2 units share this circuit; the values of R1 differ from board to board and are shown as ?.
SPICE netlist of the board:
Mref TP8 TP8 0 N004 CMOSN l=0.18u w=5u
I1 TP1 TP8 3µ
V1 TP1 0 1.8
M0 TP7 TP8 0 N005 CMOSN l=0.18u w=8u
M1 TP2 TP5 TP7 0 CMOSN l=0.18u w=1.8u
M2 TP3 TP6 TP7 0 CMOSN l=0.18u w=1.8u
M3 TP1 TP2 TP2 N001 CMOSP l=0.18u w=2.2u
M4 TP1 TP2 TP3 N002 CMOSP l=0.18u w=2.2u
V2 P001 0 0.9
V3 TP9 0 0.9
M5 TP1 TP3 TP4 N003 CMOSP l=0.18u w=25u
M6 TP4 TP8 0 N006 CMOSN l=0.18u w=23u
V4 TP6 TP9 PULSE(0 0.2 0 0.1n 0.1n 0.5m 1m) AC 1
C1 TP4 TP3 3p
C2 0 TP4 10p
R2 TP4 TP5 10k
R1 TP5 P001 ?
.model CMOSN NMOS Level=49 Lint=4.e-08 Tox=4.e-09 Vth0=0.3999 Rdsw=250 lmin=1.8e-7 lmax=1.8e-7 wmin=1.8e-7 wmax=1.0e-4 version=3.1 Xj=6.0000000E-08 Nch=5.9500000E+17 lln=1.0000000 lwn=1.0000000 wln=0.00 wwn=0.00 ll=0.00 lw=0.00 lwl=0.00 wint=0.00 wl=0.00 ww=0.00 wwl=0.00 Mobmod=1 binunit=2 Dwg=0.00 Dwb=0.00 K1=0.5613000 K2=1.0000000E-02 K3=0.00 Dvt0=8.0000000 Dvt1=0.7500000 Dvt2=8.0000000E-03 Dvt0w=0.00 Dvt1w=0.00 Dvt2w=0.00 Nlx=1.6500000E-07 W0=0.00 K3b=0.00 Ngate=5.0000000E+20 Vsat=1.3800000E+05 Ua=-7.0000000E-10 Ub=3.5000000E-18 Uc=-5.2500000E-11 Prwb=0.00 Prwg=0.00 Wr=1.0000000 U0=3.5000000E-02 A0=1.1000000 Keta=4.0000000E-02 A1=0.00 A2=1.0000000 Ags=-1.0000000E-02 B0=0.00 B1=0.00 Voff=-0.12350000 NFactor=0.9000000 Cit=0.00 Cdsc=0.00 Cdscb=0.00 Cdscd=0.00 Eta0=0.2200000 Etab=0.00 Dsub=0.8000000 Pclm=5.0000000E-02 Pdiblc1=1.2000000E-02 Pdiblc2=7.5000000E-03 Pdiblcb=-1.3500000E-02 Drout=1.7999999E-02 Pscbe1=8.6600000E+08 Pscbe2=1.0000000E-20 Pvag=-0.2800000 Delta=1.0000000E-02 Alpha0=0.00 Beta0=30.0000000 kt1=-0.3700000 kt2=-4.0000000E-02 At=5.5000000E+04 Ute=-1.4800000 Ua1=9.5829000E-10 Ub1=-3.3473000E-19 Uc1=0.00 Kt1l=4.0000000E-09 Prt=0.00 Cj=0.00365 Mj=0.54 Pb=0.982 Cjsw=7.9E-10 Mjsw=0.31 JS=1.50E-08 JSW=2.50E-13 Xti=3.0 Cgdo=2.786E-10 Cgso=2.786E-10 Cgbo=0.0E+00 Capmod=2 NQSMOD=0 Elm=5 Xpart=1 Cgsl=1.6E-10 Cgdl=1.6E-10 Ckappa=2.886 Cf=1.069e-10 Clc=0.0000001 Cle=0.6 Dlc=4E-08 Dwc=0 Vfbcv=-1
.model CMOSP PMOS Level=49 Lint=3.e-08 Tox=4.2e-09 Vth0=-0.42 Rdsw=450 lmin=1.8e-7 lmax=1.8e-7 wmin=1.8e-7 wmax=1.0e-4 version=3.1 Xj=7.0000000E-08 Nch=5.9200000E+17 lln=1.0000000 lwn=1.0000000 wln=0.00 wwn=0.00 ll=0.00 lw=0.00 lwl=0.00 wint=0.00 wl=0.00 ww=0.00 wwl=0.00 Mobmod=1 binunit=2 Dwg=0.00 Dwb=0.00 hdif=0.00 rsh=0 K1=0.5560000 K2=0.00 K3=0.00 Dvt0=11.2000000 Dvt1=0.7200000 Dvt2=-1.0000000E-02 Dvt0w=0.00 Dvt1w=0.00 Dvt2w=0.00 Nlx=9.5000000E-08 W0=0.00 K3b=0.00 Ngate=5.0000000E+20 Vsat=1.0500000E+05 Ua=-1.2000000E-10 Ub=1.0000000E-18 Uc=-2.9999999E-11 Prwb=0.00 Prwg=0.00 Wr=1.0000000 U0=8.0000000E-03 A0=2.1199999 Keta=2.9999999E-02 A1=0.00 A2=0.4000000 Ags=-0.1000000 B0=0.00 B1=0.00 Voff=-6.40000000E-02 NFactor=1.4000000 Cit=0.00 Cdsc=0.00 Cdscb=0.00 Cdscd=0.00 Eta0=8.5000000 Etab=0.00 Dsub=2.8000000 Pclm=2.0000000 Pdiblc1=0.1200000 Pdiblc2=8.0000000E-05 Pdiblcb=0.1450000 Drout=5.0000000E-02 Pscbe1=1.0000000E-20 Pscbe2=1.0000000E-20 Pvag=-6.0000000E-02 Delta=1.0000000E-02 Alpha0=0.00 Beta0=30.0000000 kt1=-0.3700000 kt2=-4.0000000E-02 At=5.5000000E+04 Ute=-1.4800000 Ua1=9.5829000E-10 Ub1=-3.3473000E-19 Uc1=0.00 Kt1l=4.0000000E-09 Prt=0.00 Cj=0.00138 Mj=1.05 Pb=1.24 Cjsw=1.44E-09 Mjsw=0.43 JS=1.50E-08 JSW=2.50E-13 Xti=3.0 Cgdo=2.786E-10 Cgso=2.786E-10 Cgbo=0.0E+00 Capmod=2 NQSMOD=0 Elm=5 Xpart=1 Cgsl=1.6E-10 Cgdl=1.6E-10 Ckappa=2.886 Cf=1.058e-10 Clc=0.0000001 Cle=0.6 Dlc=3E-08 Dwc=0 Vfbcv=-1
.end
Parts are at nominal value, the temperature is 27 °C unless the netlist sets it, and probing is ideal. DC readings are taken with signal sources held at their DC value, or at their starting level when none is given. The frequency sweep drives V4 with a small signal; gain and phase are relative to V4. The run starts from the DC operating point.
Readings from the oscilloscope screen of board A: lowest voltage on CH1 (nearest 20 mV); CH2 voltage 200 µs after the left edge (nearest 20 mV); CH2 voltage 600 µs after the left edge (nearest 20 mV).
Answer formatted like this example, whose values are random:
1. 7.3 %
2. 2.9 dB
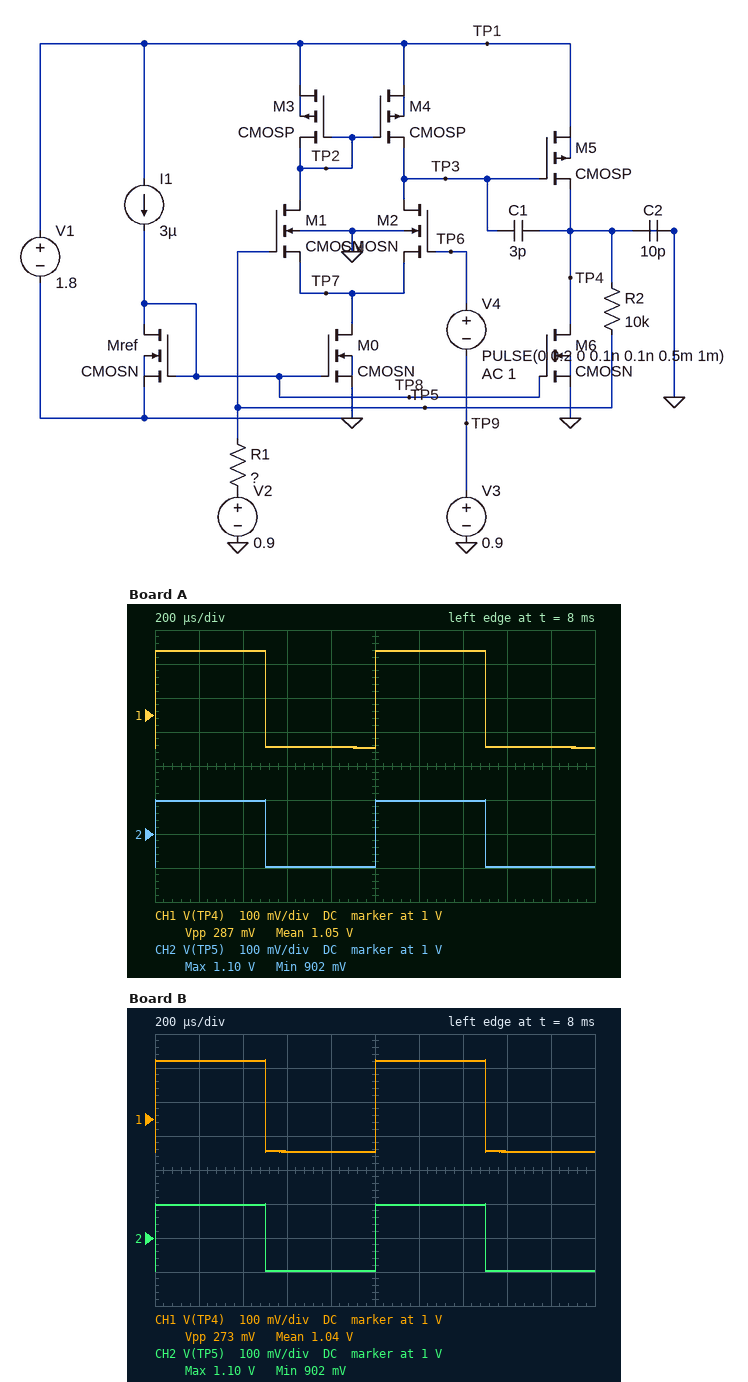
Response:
1. 900 mV
2. 1.10 V
3. 900 mV
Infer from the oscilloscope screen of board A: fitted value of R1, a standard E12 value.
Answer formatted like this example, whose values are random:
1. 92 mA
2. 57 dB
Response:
1. 22 kΩ
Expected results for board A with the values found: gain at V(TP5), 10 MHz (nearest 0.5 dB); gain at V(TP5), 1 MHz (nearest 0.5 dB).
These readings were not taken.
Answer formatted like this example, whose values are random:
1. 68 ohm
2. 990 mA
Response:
1. -13.0 dB
2. -1.0 dB
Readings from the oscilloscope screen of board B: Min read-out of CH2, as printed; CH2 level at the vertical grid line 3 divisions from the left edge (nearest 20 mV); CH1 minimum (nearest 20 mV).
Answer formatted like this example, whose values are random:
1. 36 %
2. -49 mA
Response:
1. 902 mV
2. 900 mV
3. 900 mV
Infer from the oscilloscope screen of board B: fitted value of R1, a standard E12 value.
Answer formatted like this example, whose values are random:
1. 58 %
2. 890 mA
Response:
1. 27 kΩ
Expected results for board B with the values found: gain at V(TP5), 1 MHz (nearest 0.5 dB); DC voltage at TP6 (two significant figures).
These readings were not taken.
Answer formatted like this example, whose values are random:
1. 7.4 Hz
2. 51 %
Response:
1. -0.5 dB
2. 900 mV
